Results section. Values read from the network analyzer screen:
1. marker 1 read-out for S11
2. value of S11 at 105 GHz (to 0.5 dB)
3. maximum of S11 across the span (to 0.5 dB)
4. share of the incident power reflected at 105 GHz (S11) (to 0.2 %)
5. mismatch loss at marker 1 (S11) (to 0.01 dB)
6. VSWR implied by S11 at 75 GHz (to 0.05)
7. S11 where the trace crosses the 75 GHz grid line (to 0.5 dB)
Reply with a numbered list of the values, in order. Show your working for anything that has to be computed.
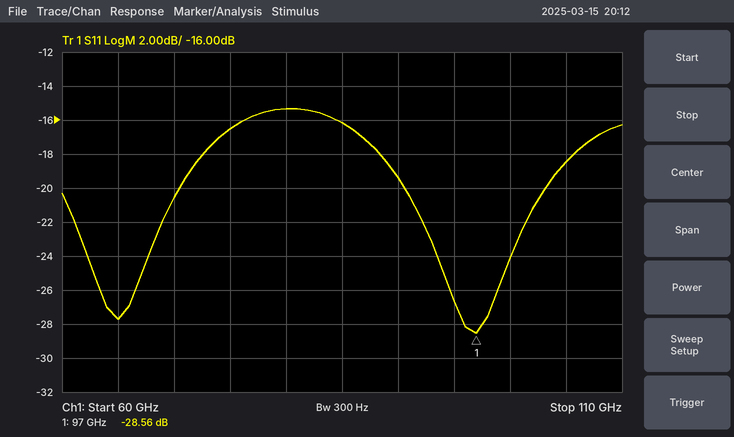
1. -28.56 dB
2. -18.5 dB
3. -15.5 dB
4. 10^(-18.5/10) ≈ 1.4 %
5. −10 log10(1 − 10^(-28.56/10)) ≈ 0.01 dB
6. |Γ| = 10^(-16.5/20) = 0.1496; VSWR = (1 + 0.1496)/(1 − 0.1496) ≈ 1.35
7. -16.5 dB
